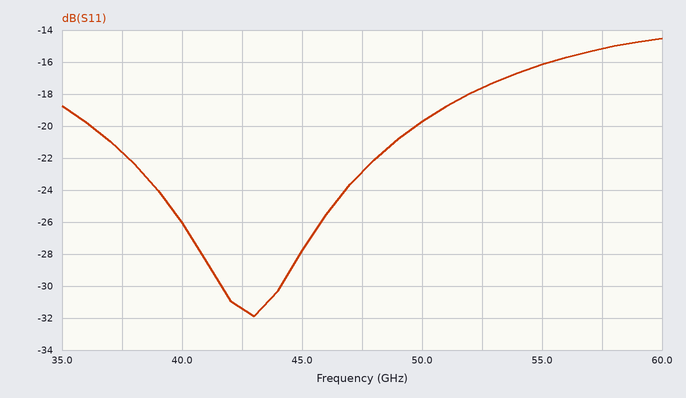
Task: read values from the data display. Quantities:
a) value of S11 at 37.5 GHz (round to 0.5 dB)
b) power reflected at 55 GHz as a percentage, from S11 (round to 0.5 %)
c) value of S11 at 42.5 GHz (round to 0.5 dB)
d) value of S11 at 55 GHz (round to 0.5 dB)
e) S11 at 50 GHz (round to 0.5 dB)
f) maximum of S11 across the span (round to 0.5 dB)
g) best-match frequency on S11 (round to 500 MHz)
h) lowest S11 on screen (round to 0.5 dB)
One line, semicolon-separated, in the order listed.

-21.5 dB; 2.5 %; -31.5 dB; -16.0 dB; -19.5 dB; -14.5 dB; 43.0 GHz; -32.0 dB
